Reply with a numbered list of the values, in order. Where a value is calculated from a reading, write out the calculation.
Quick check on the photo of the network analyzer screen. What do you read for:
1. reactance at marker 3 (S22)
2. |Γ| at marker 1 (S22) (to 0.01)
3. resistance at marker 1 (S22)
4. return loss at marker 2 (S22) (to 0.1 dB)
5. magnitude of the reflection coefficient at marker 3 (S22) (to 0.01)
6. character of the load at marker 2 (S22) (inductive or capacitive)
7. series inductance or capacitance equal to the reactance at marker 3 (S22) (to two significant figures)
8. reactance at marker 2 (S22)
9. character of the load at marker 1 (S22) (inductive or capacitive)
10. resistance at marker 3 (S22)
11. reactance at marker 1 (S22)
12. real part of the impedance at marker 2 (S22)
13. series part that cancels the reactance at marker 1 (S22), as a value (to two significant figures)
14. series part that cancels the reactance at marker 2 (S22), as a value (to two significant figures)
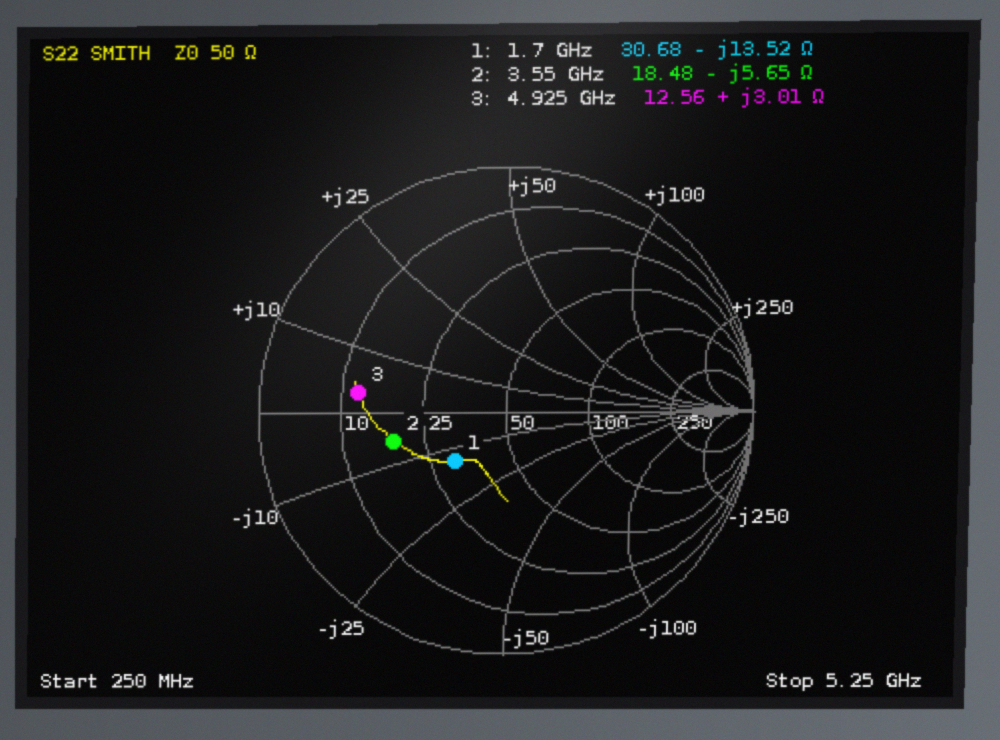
1. +3.01 Ω
2. 0.29
3. 30.68 Ω
4. 6.6 dB
5. 0.60
6. capacitive
7. L = 3.01 Ω/(2π × 4.925 GHz) ≈ 97 pH
8. -5.65 Ω
9. capacitive
10. 12.56 Ω
11. -13.52 Ω
12. 18.48 Ω
13. L = 13.52 Ω/(2π × 1.7 GHz) ≈ 1.3 nH
14. L = 5.65 Ω/(2π × 3.55 GHz) ≈ 253 pH, so 250 pH to two significant figures
